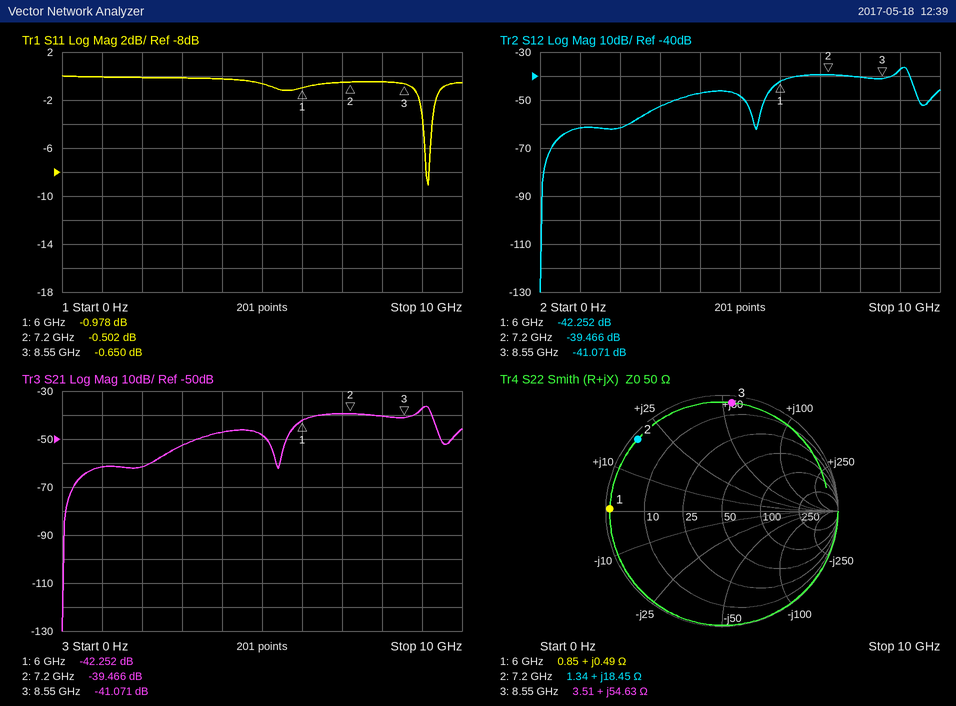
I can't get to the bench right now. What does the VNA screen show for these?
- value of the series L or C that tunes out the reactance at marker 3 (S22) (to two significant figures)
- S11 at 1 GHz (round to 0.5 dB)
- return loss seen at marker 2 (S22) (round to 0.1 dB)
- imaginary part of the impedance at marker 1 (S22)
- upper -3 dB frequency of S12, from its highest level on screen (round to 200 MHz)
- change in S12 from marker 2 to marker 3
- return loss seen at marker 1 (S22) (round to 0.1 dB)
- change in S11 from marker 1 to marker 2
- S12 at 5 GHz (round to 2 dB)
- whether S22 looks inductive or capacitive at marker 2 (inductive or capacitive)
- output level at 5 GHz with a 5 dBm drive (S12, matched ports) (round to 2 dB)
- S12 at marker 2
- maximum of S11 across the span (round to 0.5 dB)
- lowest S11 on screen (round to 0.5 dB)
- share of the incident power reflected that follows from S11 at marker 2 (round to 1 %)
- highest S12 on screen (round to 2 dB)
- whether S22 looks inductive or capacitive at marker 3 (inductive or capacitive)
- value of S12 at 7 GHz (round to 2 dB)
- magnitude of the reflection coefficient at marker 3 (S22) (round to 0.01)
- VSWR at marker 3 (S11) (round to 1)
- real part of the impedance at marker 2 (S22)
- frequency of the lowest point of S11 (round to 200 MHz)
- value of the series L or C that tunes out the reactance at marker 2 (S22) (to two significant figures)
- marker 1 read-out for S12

340 fF
0.0 dB
0.4 dB
+0.49 Ω
9.2 GHz
-1.605 dB
0.3 dB
0.476 dB
-48 dB
inductive
-44 dBm
-39.466 dB
0.0 dB
-9.0 dB
89 %
-36 dB
inductive
-40 dB
0.94
27
1.34 Ω
9.2 GHz
1.2 pF
-42.252 dB
